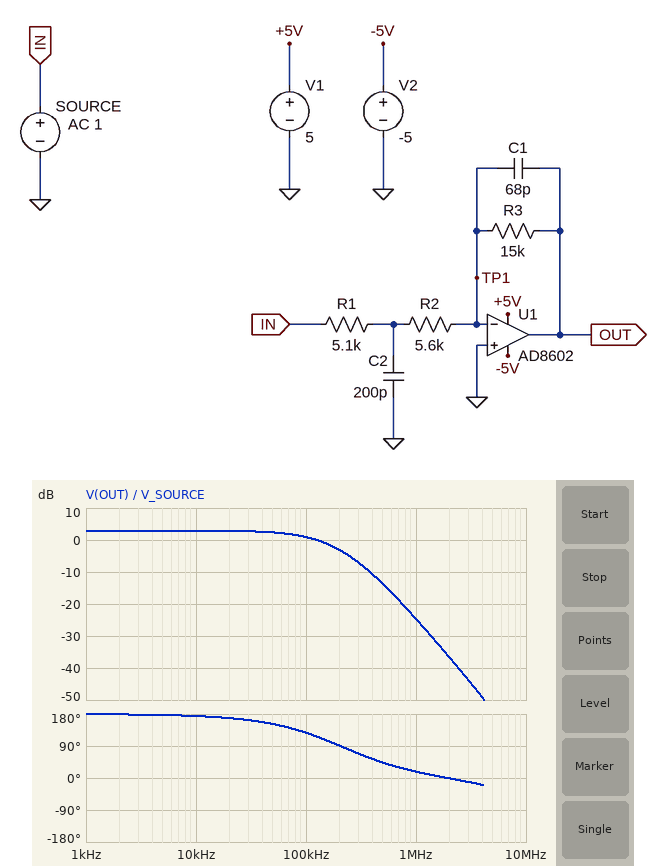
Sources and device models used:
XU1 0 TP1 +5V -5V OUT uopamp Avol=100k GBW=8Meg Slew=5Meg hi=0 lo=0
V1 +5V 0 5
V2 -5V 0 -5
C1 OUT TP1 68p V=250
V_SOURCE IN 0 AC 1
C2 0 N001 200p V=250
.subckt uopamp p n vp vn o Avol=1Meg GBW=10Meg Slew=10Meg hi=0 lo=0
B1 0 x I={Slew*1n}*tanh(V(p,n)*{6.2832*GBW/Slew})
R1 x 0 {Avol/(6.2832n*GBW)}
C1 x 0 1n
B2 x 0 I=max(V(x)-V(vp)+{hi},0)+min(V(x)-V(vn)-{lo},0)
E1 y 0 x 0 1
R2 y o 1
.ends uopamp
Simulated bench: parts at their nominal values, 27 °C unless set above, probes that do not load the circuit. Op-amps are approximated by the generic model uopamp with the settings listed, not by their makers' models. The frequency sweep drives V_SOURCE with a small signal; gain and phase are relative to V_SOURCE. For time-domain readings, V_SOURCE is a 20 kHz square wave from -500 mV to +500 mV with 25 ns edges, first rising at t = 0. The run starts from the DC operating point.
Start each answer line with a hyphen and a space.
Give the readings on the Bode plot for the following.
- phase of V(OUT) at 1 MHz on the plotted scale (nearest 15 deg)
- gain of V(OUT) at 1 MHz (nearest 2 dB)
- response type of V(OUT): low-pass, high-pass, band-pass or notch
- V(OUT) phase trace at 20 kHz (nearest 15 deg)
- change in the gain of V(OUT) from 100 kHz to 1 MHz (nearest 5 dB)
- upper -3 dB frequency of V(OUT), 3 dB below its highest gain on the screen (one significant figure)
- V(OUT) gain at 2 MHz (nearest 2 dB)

- 15 deg
- -24 dB
- low-pass
- 165 deg
- -25 dB
- 100 kHz
- -36 dB
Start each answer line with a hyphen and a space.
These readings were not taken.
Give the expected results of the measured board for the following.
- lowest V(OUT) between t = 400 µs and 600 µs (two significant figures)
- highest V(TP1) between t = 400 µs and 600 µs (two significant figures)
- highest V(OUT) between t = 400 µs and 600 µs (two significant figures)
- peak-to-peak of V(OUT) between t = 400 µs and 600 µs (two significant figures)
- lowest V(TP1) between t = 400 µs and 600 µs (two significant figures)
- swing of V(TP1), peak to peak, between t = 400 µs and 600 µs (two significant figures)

- -700 mV
- 13 mV
- 700 mV
- 1.4 V
- -13 mV
- 27 mV
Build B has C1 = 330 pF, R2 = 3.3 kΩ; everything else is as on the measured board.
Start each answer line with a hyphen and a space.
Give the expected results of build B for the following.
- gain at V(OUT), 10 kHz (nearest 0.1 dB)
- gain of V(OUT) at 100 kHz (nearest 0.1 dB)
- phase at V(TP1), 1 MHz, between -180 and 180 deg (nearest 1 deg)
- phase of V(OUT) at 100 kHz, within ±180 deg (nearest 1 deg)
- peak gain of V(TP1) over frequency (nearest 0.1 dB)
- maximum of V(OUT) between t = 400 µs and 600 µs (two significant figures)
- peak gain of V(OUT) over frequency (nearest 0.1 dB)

- 4.6 dB
- -5.6 dB
- -74 deg
- 93 deg
- -43.6 dB
- 880 mV
- 5.0 dB
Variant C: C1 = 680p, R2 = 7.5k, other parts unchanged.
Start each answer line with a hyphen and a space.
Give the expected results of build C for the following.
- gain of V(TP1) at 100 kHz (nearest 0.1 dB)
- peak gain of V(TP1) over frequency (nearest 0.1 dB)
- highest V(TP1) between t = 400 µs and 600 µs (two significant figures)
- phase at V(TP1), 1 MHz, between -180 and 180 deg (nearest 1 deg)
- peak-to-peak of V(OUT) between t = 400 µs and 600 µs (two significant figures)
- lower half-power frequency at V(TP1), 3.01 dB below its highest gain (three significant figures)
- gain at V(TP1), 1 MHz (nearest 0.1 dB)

- -53.4 dB
- -53.2 dB
- 1.8 mV
- -81 deg
- 990 mV
- 14.0 kHz
- -64.7 dB
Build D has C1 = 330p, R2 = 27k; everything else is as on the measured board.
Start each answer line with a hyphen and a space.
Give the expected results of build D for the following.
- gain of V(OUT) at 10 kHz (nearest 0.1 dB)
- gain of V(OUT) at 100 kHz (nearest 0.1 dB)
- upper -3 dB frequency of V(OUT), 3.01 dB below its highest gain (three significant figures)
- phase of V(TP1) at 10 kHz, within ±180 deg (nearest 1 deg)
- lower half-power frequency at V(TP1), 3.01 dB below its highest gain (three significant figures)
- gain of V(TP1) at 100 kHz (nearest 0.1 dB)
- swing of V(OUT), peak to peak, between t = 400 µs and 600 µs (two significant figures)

- -7.0 dB
- -18.0 dB
- 31.2 kHz
- 69 deg
- 24.6 kHz
- -56.1 dB
- 460 mV
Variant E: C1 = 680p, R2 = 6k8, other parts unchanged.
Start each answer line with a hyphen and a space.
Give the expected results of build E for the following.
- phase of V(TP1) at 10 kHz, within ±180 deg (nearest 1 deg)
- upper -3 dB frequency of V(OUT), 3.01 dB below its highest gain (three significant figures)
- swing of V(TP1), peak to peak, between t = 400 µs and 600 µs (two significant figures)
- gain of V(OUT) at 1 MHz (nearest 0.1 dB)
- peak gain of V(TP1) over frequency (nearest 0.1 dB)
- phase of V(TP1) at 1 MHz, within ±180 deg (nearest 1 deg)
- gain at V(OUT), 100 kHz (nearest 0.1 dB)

- 55 deg
- 15.5 kHz
- 3.8 mV
- -45.8 dB
- -52.7 dB
- -81 deg
- -14.8 dB
